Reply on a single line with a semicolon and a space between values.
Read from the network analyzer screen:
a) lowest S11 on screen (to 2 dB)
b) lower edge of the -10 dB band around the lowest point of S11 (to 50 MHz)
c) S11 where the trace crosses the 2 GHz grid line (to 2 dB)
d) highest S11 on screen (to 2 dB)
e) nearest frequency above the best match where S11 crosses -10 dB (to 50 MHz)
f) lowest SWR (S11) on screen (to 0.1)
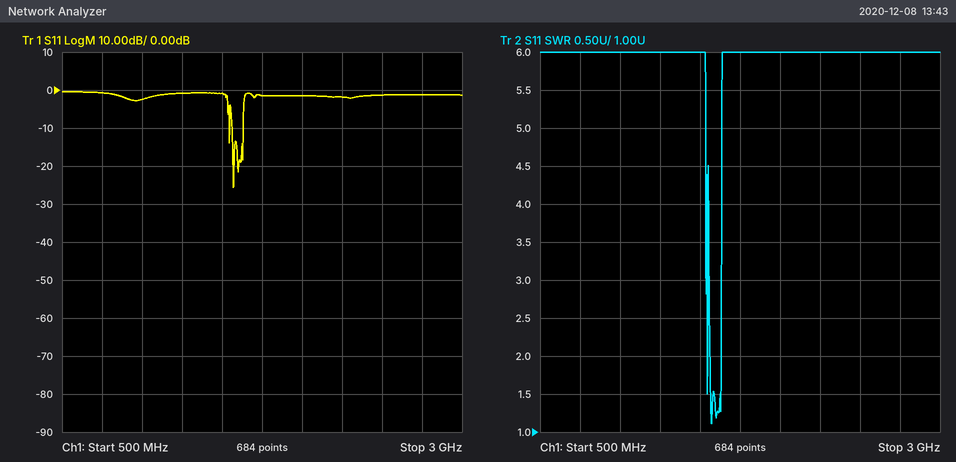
-26 dB; 1.55 GHz; -2 dB; 0 dB; 1.65 GHz; 1.1
